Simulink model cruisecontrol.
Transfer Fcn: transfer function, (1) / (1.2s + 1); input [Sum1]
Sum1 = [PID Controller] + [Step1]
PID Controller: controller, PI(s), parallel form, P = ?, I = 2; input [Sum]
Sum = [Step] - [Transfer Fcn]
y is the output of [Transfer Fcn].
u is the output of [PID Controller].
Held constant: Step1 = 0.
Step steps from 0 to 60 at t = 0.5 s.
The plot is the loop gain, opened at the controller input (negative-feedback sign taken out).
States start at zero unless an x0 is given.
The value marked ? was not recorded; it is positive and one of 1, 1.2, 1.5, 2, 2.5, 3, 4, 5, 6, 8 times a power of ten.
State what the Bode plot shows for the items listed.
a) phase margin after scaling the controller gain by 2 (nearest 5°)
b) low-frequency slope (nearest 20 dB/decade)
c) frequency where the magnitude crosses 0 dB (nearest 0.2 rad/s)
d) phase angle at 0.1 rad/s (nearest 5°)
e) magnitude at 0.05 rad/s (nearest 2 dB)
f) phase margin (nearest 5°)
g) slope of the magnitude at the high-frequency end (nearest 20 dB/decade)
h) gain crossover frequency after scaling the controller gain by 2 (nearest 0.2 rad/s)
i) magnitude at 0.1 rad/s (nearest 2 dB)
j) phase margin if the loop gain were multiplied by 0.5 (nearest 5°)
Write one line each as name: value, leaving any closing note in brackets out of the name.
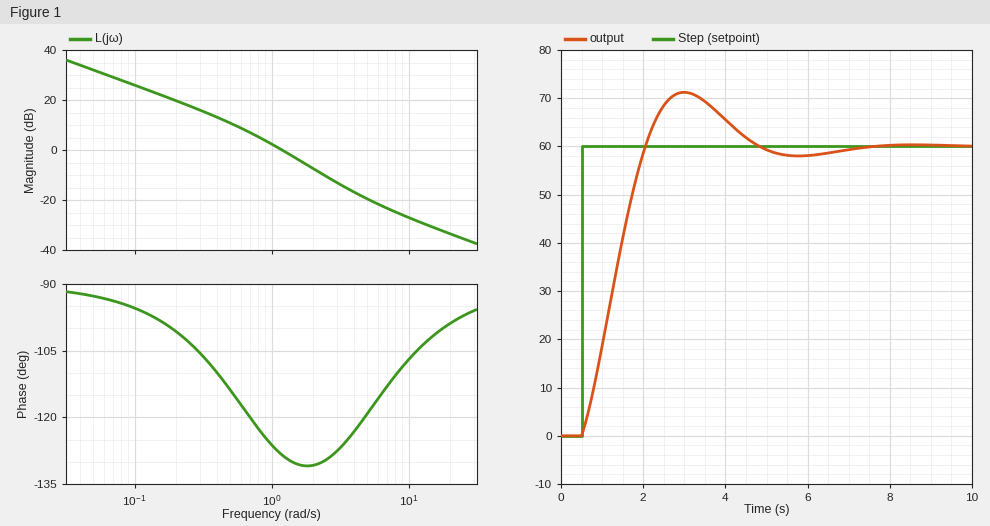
phase margin after scaling the controller gain by 2: 50°
low-frequency slope: -20 dB/decade
frequency where the magnitude crosses 0 dB: 1.2 rad/s
phase angle at 0.1 rad/s: -95°
magnitude at 0.05 rad/s: 32 dB
phase margin: 50°
slope of the magnitude at the high-frequency end: -20 dB/decade
gain crossover frequency after scaling the controller gain by 2: 1.8 rad/s
magnitude at 0.1 rad/s: 26 dB
phase margin if the loop gain were multiplied by 0.5: 60°
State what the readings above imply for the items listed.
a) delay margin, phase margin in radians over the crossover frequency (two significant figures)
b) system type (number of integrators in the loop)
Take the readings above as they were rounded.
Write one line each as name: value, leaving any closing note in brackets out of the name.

delay margin, phase margin in radians over the crossover frequency: 0.73 s
system type: 1
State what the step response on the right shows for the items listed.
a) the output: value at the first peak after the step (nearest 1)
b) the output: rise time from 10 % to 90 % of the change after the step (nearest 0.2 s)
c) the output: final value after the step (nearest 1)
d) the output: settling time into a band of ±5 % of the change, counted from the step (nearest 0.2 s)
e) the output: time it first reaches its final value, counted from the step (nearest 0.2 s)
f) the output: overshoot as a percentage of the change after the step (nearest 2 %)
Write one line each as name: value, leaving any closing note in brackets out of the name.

the output: value at the first peak after the step: 71
the output: rise time from 10 % to 90 % of the change after the step: 1.2 s
the output: final value after the step: 60
the output: settling time into a band of ±5 % of the change, counted from the step: 3.8 s
the output: time it first reaches its final value, counted from the step: 1.6 s
the output: overshoot as a percentage of the change after the step: 18 %
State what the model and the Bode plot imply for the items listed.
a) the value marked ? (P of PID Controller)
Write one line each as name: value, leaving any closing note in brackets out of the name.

the value marked ?: 0.5
